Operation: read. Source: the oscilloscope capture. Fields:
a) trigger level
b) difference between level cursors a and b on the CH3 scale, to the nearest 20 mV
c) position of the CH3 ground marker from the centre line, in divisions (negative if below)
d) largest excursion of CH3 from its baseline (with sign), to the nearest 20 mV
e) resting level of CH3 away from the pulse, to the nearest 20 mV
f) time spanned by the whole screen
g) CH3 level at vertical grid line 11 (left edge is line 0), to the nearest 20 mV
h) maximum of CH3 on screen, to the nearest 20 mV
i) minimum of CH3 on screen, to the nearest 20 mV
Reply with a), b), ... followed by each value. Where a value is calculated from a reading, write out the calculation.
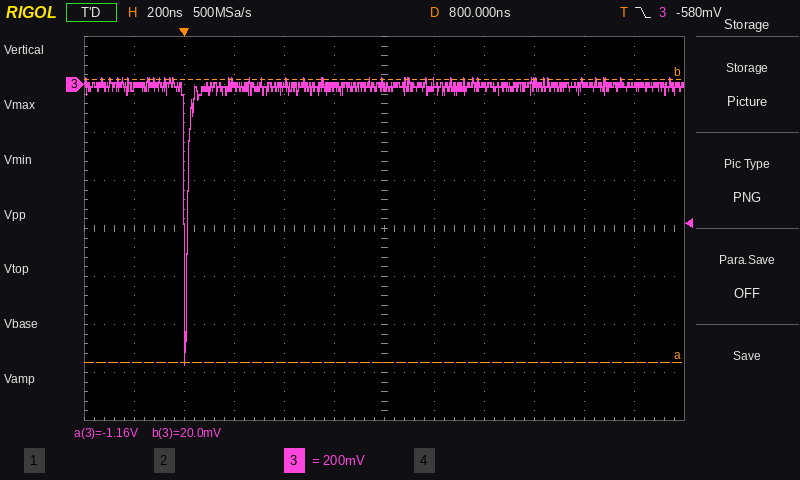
a) -580 mV
b) 1.18 V
c) +3.0 div
d) -1.16 V − (0 mV) = -1.16 V
e) 0 mV
f) 2.4 µs
g) 0 mV
h) 20 mV
i) -1.16 V
